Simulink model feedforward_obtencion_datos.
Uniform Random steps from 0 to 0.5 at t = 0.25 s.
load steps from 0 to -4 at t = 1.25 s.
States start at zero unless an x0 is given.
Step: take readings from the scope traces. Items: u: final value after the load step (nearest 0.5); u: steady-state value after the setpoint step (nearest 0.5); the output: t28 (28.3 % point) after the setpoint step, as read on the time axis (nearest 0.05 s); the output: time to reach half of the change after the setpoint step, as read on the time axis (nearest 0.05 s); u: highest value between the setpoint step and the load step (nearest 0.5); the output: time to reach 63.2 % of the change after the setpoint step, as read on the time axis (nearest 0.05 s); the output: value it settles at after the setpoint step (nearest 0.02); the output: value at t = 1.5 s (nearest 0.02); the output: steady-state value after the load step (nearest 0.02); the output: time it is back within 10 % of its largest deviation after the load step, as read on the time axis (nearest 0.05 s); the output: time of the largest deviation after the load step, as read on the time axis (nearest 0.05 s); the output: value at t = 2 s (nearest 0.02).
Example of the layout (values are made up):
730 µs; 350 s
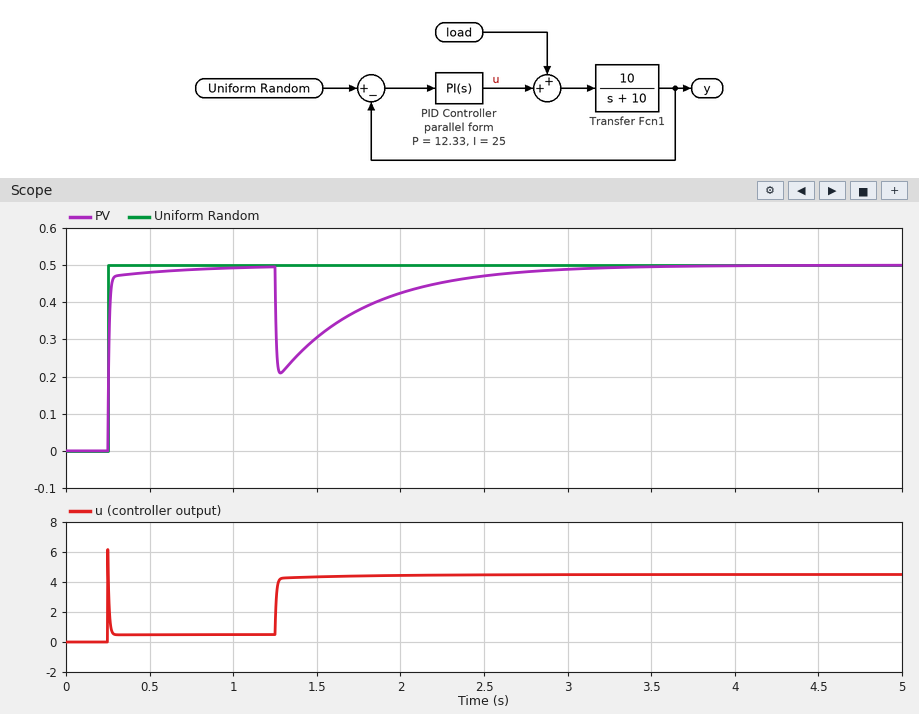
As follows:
4.5; 0.5; 0.25 s; 0.25 s; 6.0; 0.25 s; 0.50; 0.30; 0.50; 2.50 s; 1.30 s; 0.42
